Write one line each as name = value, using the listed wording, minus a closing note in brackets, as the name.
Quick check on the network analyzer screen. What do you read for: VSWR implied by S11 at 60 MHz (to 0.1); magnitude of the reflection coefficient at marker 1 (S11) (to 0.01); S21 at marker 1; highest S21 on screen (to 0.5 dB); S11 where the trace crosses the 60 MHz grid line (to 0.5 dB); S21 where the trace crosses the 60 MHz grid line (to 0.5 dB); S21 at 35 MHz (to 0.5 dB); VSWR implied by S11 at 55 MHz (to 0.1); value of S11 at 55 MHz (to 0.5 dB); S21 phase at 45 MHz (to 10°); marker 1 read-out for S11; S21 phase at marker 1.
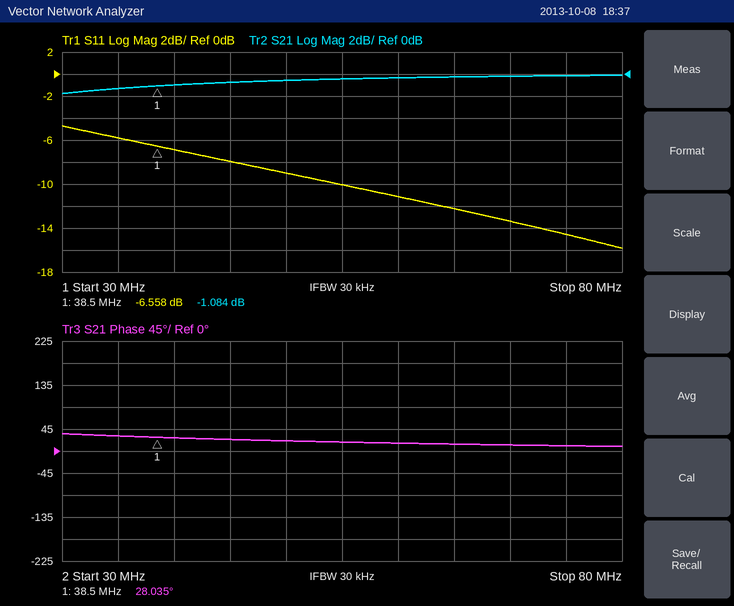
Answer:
VSWR implied by S11 at 60 MHz = 1.8
magnitude of the reflection coefficient at marker 1 (S11) = 0.47
S21 at marker 1 = -1.084 dB
highest S21 on screen = 0.0 dB
S11 where the trace crosses the 60 MHz grid line = -11.0 dB
S21 where the trace crosses the 60 MHz grid line = -0.5 dB
S21 at 35 MHz = -1.5 dB
VSWR implied by S11 at 55 MHz = 1.9
value of S11 at 55 MHz = -10.0 dB
S21 phase at 45 MHz = 20°
marker 1 read-out for S11 = -6.558 dB
S21 phase at marker 1 = 28.035°
